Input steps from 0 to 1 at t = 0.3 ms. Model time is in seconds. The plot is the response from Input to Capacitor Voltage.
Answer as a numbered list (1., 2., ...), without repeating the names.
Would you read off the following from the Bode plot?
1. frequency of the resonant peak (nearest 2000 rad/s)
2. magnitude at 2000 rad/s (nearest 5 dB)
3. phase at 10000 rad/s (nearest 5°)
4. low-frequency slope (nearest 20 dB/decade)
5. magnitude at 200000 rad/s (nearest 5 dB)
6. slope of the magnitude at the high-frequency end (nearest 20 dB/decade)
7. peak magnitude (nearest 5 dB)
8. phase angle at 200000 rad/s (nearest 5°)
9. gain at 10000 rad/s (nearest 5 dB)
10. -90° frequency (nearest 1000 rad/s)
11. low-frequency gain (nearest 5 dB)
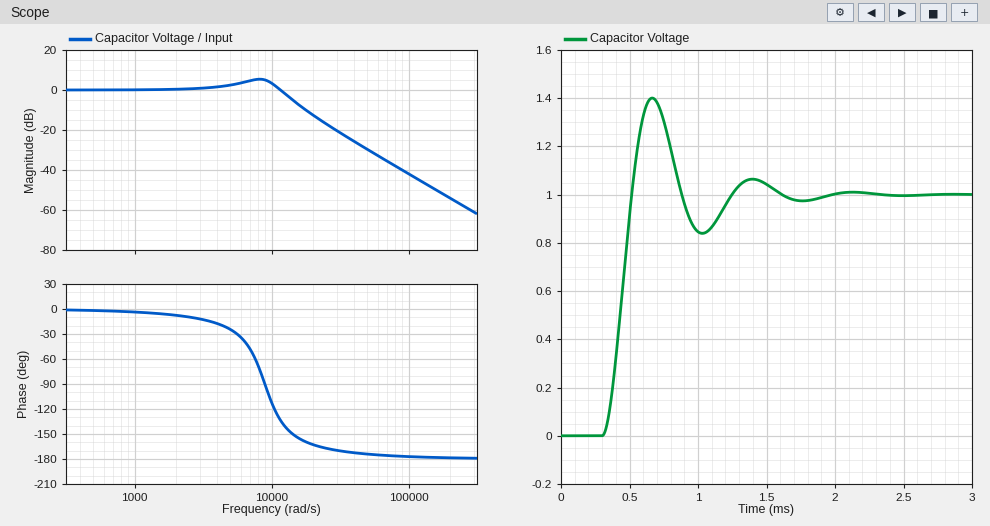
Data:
1. 8000 rad/s
2. 0 dB
3. -110°
4. 0 dB/decade
5. -55 dB
6. -40 dB/decade
7. 5 dB
8. -180°
9. 5 dB
10. 9000 rad/s
11. 0 dB
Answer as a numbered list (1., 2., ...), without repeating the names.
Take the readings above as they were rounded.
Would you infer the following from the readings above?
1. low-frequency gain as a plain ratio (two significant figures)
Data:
1. 1.0
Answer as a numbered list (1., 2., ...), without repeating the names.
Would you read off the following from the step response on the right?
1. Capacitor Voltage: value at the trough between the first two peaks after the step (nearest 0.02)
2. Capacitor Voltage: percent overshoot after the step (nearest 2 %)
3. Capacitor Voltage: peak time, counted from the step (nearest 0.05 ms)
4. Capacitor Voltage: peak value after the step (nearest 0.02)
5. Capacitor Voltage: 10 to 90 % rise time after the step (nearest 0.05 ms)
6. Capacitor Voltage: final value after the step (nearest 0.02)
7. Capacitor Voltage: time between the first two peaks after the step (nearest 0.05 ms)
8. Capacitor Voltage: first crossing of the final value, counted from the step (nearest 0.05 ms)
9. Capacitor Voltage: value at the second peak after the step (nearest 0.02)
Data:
1. 0.84
2. 40 %
3. 0.35 ms
4. 1.40
5. 0.15 ms
6. 1.00
7. 0.75 ms
8. 0.20 ms
9. 1.06
